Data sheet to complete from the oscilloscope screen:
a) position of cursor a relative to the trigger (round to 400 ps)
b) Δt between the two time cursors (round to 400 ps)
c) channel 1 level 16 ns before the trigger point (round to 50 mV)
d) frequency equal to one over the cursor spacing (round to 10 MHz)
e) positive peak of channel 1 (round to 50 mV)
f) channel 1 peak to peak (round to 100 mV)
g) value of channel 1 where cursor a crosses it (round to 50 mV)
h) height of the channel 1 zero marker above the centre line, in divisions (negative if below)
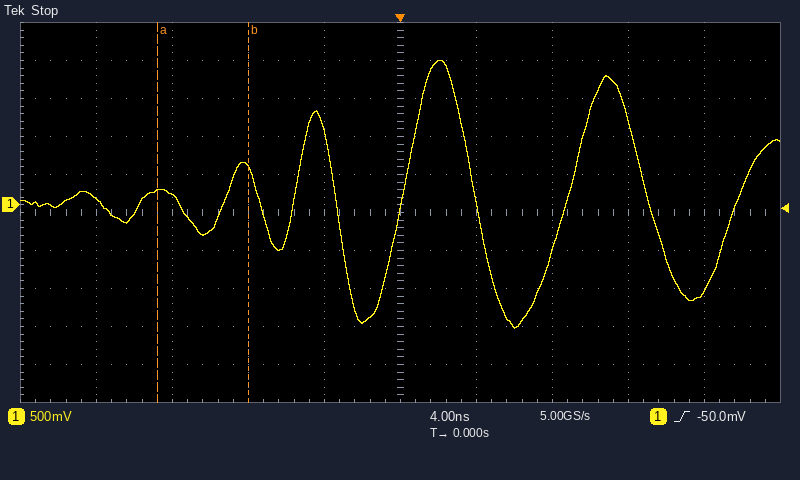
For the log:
-12.8 ns
4.8 ns
100 mV
210 MHz
1.90 V
3.50 V
200 mV
+0.2 div
